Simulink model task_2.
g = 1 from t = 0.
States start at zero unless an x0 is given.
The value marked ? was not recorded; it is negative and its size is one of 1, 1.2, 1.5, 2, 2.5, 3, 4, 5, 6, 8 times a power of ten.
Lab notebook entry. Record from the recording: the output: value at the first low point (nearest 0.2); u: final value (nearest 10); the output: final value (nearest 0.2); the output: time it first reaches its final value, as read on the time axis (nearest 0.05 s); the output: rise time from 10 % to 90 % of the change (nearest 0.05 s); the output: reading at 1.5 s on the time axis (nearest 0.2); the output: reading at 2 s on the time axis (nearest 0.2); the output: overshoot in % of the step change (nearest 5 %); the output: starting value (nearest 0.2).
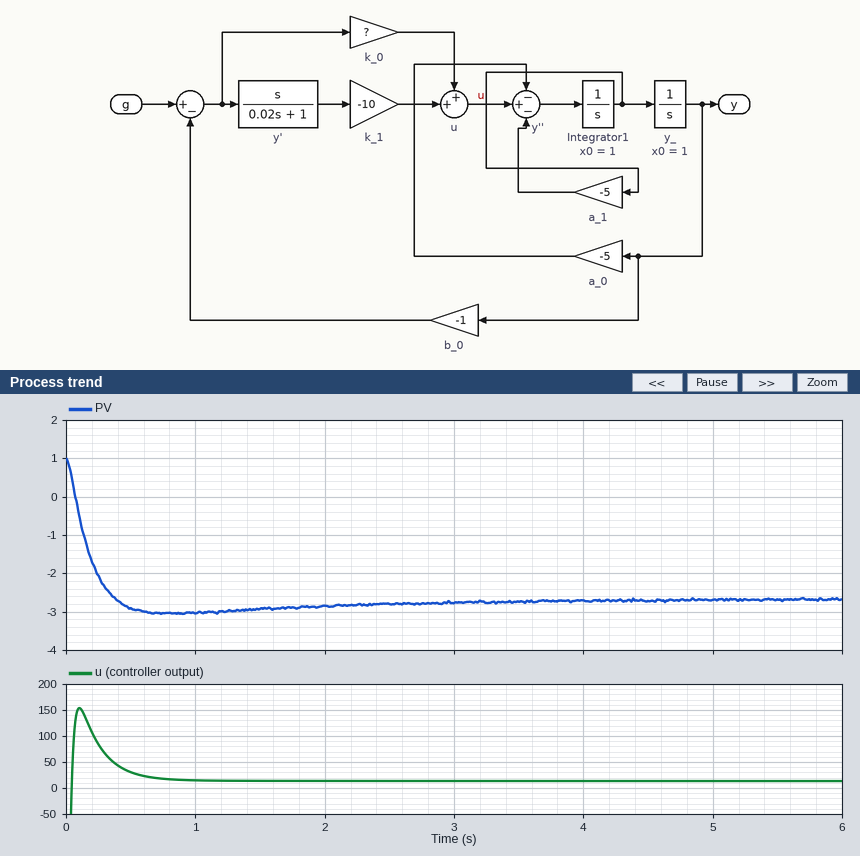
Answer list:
-3.0
10
-2.6
0.40 s
0.25 s
-3.0
-2.8
10 %
1.0
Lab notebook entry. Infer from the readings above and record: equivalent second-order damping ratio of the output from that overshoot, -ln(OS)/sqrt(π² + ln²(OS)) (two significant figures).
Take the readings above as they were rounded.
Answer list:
0.59
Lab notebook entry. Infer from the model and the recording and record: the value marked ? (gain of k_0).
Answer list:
-8
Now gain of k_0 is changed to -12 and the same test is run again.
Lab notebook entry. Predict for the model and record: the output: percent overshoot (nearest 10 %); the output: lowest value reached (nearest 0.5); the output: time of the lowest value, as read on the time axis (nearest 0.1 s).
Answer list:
40 %
-3.0
0.5 s
